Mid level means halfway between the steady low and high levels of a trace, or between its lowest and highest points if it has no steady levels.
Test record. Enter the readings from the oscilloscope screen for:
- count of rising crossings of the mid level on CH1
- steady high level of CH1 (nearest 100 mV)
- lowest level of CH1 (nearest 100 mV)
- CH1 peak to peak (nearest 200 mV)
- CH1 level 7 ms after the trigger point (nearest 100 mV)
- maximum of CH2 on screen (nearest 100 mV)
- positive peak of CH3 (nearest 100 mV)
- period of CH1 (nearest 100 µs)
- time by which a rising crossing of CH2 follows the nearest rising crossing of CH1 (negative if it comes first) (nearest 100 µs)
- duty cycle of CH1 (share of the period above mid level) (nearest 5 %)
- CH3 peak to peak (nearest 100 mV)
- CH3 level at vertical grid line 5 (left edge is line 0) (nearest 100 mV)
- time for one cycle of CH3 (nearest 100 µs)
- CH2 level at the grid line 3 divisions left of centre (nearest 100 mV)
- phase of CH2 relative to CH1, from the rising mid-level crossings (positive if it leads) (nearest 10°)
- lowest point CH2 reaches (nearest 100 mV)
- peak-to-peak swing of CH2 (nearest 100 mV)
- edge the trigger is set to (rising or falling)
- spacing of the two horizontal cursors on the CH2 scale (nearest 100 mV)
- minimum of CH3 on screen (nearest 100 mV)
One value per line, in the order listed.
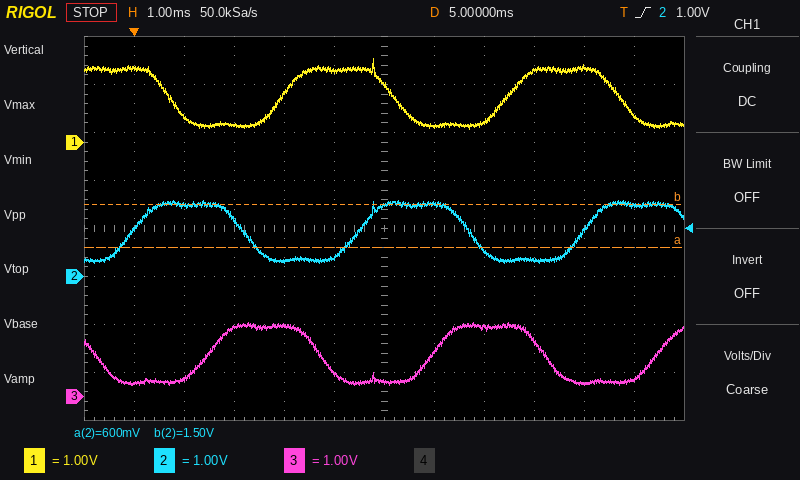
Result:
2
1.5 V
300 mV
1.4 V
400 mV
1.6 V
1.5 V
4.5 ms
+1.5 ms
50 %
1.3 V
500 mV
4.5 ms
1.2 V
-120°
300 mV
1.3 V
rising
900 mV
200 mV
